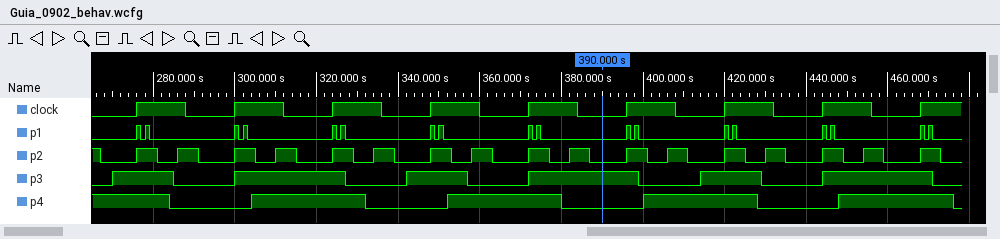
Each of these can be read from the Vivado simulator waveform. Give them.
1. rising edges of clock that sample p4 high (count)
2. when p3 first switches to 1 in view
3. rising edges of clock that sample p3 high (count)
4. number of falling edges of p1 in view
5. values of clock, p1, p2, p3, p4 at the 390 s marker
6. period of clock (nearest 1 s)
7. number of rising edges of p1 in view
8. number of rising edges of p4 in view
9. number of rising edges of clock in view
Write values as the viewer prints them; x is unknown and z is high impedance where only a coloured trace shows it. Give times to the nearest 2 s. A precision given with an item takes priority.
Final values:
5
270 s
6
18
clock=0, p1=0, p2=0, p3=1, p4=0
24 s
18
4
9
